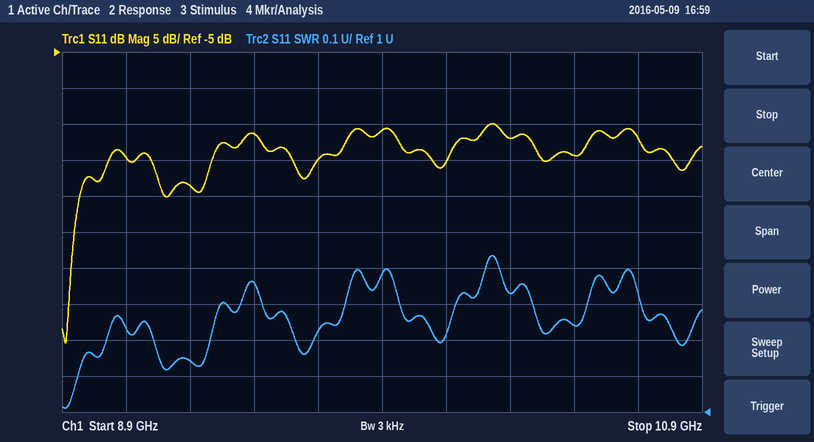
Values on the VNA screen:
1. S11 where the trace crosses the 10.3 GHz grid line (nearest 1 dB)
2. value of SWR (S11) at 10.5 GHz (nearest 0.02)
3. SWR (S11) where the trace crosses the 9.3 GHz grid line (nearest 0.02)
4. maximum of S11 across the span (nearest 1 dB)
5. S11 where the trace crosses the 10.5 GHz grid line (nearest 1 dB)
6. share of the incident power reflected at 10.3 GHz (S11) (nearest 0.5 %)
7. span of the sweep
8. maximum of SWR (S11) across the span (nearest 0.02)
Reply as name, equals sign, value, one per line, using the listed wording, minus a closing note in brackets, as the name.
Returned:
S11 where the trace crosses the 10.3 GHz grid line = -17 dB
value of SWR (S11) at 10.5 GHz = 1.24
SWR (S11) where the trace crosses the 9.3 GHz grid line = 1.14
maximum of S11 across the span = -15 dB
S11 where the trace crosses the 10.5 GHz grid line = -19 dB
share of the incident power reflected at 10.3 GHz (S11) = 2.0 %
span of the sweep = 2 GHz
maximum of SWR (S11) across the span = 1.44
